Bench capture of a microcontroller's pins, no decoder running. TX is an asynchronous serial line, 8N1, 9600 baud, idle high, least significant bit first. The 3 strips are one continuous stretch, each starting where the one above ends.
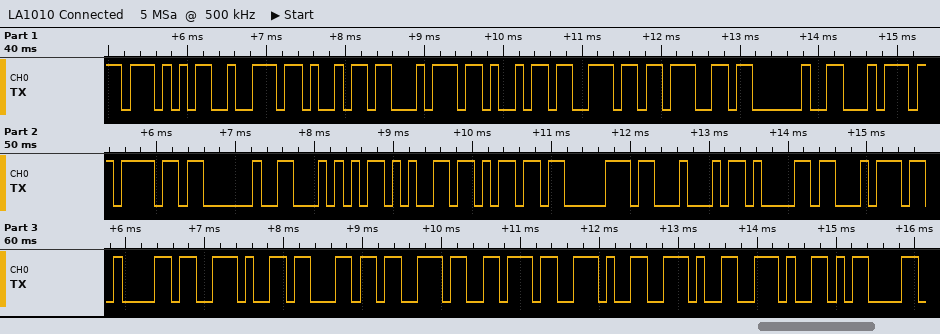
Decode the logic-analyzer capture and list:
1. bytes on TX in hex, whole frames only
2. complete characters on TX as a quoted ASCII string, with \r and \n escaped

57 72 69 74 69 6E 67 20 74 6F 20 54 65 6D 70 44 61 74 61 2E 63 73 76 2E 2E 2E 0D
"Writing to TempData.csv...\r"
